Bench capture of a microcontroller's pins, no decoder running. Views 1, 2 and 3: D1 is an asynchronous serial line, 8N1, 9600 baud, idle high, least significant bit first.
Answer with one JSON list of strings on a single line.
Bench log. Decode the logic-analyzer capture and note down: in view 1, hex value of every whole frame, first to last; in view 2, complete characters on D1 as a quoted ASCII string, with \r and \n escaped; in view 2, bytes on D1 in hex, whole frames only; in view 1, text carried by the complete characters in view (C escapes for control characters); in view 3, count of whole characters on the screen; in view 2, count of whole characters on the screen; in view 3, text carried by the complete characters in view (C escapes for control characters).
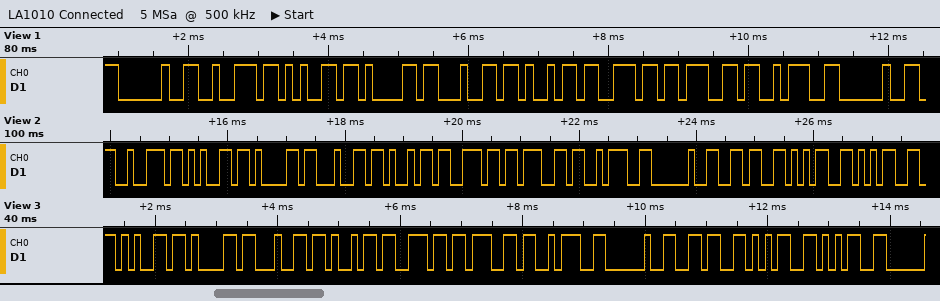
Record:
["20 72 65 61 64 69 6E 67 3A 20", "\"reading: 655\"", "72 65 61 64 69 6E 67 3A 20 36 35 35", "\" reading: \"", "11", "12", "\"eading: 655\""]
